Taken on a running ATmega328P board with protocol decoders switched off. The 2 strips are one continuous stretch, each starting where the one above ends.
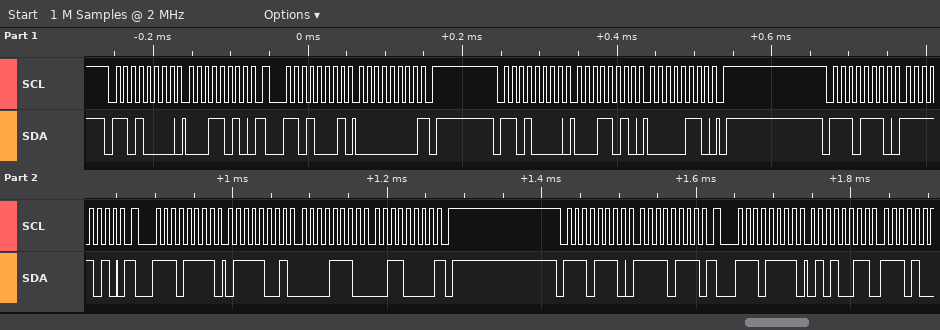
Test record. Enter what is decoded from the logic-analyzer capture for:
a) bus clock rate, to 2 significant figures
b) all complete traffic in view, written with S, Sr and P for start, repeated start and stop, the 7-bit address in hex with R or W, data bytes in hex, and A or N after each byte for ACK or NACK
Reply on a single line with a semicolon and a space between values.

100 kHz; S 68W A 1A A Sr 68R A 00 N P S 68W A 1A A 06 A P S 77W A FA A Sr 77R A 79 A 0E A 30 N P S 77W A F7 A Sr 77R A 53 A
